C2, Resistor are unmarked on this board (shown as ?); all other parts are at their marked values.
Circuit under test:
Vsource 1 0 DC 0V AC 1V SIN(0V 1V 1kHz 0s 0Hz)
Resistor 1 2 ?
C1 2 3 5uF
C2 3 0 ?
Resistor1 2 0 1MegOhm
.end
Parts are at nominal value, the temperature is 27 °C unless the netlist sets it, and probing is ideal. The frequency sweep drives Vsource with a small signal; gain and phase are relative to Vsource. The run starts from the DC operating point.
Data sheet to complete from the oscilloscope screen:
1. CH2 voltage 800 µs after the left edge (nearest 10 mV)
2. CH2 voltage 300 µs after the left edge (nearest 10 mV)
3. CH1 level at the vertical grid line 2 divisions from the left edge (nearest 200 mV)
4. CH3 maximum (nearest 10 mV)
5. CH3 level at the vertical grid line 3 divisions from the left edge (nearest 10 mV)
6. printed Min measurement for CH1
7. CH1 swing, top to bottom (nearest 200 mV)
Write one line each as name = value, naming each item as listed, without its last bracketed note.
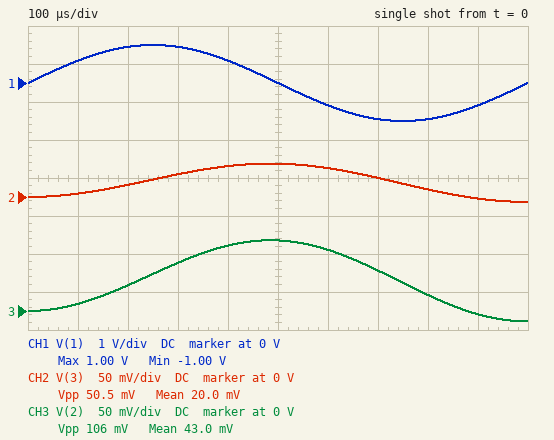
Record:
CH2 voltage 800 µs after the left edge = 10 mV
CH2 voltage 300 µs after the left edge = 30 mV
CH1 level at the vertical grid line 2 divisions from the left edge = 1.0 V
CH3 maximum = 90 mV
CH3 level at the vertical grid line 3 divisions from the left edge = 60 mV
printed Min measurement for CH1 = -1.00 V
CH1 swing, top to bottom = 2.0 V
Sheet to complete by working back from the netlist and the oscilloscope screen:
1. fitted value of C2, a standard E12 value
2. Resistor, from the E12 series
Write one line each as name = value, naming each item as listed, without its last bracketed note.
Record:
fitted value of C2, a standard E12 value = 5.6 µF
Resistor, from the E12 series = 1.2 kΩ
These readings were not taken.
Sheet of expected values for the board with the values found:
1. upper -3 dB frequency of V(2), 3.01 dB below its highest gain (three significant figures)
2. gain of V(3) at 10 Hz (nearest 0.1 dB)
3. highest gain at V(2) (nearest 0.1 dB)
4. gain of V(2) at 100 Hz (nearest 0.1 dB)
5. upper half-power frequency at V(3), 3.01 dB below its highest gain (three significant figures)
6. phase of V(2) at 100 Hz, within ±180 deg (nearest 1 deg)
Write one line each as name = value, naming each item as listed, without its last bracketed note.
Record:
upper -3 dB frequency of V(2), 3.01 dB below its highest gain = 50.3 Hz
gain of V(3) at 10 Hz = -6.7 dB
highest gain at V(2) = 0 dB
gain of V(2) at 100 Hz = -7.0 dB
upper half-power frequency at V(3), 3.01 dB below its highest gain = 50.3 Hz
phase of V(2) at 100 Hz, within ±180 deg = -63 deg
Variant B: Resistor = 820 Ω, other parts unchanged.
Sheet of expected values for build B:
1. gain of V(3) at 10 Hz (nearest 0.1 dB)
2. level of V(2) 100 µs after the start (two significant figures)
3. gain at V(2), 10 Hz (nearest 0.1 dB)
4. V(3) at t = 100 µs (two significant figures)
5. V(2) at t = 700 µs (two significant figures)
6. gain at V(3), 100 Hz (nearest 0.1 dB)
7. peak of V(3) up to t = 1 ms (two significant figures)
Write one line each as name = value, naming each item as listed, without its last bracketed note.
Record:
gain of V(3) at 10 Hz = -6.6 dB
level of V(2) 100 µs after the start = 14 mV
gain at V(2), 10 Hz = -0.1 dB
V(3) at t = 100 µs = 6.5 mV
V(2) at t = 700 µs = 70 mV
gain at V(3), 100 Hz = -11.1 dB
peak of V(3) up to t = 1 ms = 62 mV
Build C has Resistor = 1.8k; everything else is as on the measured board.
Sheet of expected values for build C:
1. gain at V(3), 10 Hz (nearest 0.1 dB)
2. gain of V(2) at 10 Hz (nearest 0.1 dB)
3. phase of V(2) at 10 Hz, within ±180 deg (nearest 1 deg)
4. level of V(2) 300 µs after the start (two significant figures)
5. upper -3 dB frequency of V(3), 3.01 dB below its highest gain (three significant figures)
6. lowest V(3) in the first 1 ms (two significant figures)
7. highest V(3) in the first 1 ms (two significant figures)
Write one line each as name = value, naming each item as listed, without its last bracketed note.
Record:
gain at V(3), 10 Hz = -6.9 dB
gain of V(2) at 10 Hz = -0.4 dB
phase of V(2) at 10 Hz, within ±180 deg = -17 deg
level of V(2) 300 µs after the start = 43 mV
upper -3 dB frequency of V(3), 3.01 dB below its highest gain = 33.5 Hz
lowest V(3) in the first 1 ms = -3.0 mV
highest V(3) in the first 1 ms = 30 mV
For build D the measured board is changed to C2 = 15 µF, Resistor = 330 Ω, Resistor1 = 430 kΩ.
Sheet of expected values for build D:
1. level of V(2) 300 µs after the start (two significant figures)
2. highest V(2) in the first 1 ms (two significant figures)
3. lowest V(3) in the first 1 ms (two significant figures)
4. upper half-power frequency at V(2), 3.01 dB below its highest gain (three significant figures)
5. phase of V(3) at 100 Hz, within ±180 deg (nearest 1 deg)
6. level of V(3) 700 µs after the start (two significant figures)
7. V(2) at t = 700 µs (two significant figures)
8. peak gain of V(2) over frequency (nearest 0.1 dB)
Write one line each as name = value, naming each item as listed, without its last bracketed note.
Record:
level of V(2) 300 µs after the start = 150 mV
highest V(2) in the first 1 ms = 210 mV
lowest V(3) in the first 1 ms = -18 mV
upper half-power frequency at V(2), 3.01 dB below its highest gain = 129 Hz
phase of V(3) at 100 Hz, within ±180 deg = -38 deg
level of V(3) 700 µs after the start = 24 mV
V(2) at t = 700 µs = 95 mV
peak gain of V(2) over frequency = 0 dB
